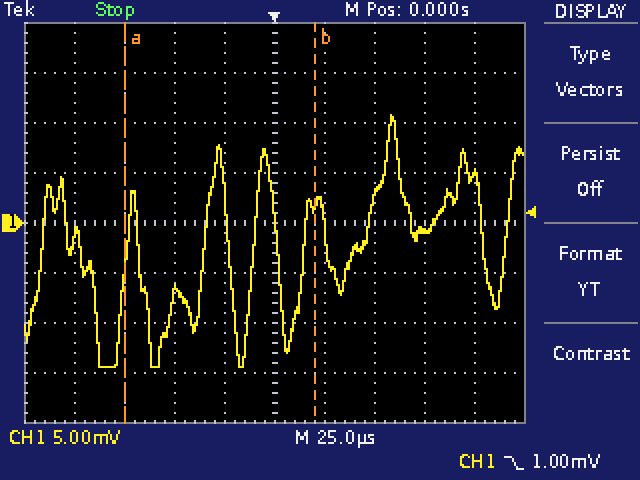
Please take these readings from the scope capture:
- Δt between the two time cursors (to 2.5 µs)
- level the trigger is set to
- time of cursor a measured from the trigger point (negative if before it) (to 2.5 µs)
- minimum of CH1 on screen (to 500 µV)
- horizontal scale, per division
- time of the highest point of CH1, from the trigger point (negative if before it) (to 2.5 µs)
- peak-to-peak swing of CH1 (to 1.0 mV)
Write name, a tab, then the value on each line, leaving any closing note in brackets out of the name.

Δt between the two time cursors	95.0 µs
level the trigger is set to	1.00 mV
time of cursor a measured from the trigger point (negative if before it)	-75.0 µs
minimum of CH1 on screen	-14.5 mV
horizontal scale, per division	25 µs
time of the highest point of CH1, from the trigger point (negative if before it)	+60.0 µs
peak-to-peak swing of CH1	25.0 mV
